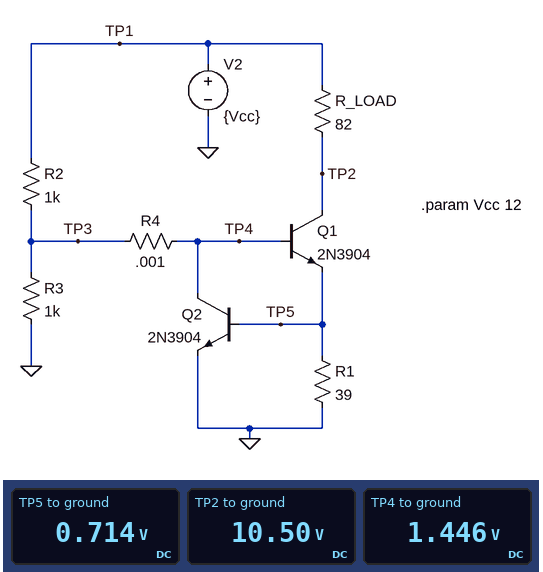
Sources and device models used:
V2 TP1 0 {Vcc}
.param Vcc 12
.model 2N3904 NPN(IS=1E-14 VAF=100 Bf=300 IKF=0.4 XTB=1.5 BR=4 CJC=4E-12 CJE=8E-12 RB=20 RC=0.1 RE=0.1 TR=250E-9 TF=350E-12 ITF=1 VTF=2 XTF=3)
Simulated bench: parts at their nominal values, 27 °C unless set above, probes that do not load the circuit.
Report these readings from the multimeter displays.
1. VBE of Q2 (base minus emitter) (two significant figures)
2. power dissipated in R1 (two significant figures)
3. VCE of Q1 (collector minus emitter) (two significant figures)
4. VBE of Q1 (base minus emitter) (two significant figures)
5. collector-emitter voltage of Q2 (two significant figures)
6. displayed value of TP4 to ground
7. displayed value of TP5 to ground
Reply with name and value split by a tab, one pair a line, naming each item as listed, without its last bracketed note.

VBE of Q2 (base minus emitter)	710 mV
power dissipated in R1	13 mW
VCE of Q1 (collector minus emitter)	9.8 V
VBE of Q1 (base minus emitter)	730 mV
collector-emitter voltage of Q2	1.4 V
displayed value of TP4 to ground	1.446 V
displayed value of TP5 to ground	0.714 V
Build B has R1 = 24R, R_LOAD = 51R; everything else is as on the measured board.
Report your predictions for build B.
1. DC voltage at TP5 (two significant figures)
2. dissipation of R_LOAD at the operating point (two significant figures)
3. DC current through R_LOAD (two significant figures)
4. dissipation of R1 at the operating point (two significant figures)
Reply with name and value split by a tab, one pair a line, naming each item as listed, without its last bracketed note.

DC voltage at TP5	710 mV
dissipation of R_LOAD at the operating point	45 mW
DC current through R_LOAD	30 mA
dissipation of R1 at the operating point	21 mW
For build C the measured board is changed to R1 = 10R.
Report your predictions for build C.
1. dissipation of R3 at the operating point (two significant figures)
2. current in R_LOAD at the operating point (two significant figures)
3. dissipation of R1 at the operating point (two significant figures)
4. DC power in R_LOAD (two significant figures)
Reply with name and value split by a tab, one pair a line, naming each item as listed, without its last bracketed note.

dissipation of R3 at the operating point	2.2 mW
current in R_LOAD at the operating point	71 mA
dissipation of R1 at the operating point	51 mW
DC power in R_LOAD	410 mW
